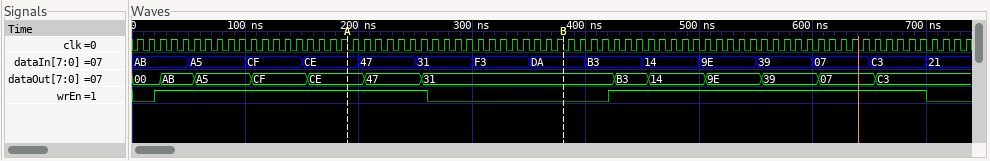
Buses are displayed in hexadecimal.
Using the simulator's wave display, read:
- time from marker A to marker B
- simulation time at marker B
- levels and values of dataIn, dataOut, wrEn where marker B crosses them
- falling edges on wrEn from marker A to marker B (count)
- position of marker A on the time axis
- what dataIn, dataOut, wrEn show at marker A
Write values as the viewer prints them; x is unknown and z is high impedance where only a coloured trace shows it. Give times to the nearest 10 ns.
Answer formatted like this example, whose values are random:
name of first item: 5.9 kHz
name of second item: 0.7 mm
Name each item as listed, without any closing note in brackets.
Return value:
time from marker A to marker B: 190 ns
simulation time at marker B: 380 ns
levels and values of dataIn, dataOut, wrEn where marker B crosses them: dataIn=DA, dataOut=31, wrEn=0
falling edges on wrEn from marker A to marker B: 1
position of marker A on the time axis: 190 ns
what dataIn, dataOut, wrEn show at marker A: dataIn=CE, dataOut=CE, wrEn=1
